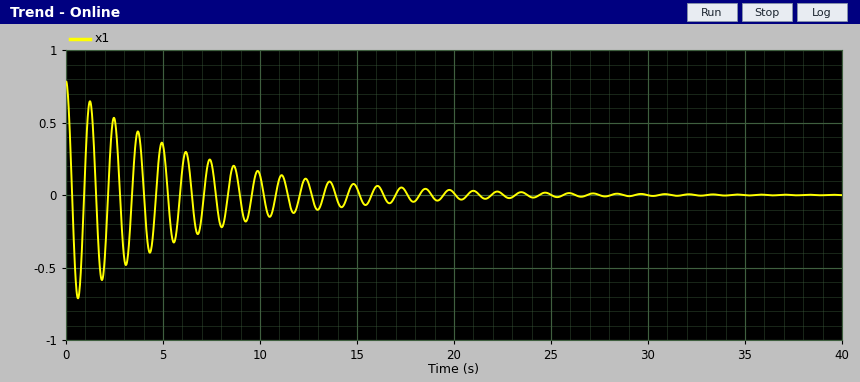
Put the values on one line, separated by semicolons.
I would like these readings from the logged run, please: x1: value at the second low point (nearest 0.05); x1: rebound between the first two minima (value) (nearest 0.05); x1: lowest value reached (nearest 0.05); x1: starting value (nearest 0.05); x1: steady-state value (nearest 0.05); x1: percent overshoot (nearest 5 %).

-0.60; 0.65; -0.70; 0.80; 0.00; 90 %
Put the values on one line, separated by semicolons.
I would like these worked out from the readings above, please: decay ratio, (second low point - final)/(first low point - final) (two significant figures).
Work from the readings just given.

0.86
